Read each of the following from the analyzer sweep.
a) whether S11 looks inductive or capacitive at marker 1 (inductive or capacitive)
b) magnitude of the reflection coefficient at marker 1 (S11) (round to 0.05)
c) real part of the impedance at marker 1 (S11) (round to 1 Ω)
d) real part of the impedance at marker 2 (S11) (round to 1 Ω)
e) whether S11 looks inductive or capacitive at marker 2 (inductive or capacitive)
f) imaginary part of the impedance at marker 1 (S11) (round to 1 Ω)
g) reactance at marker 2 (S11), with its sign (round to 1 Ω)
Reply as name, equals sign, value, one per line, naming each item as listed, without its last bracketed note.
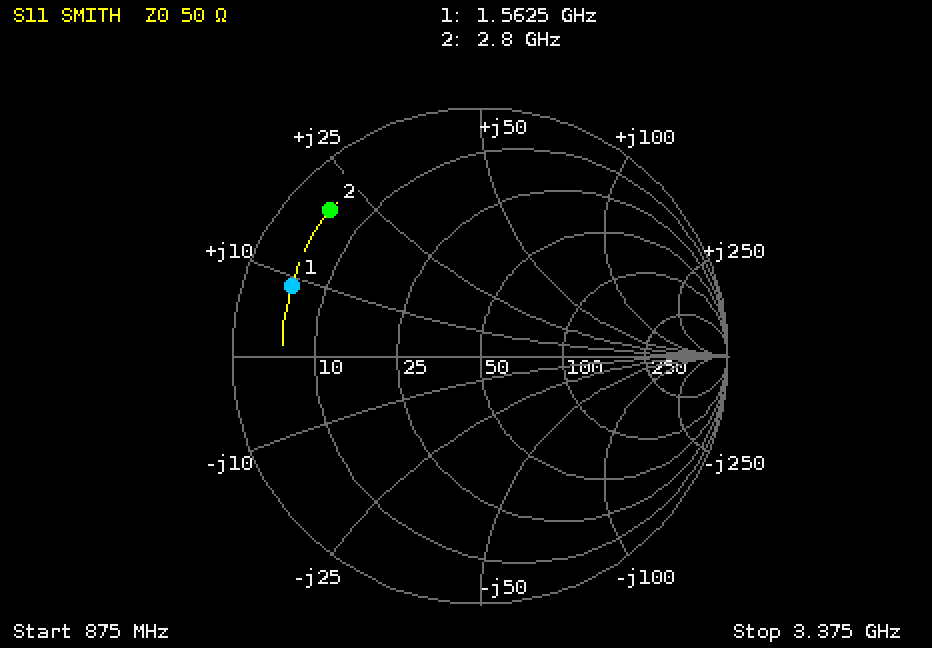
whether S11 looks inductive or capacitive at marker 1 = inductive
magnitude of the reflection coefficient at marker 1 (S11) = 0.80
real part of the impedance at marker 1 (S11) = 5 Ω
real part of the impedance at marker 2 (S11) = 5 Ω
whether S11 looks inductive or capacitive at marker 2 = inductive
imaginary part of the impedance at marker 1 (S11) = +9 Ω
reactance at marker 2 (S11), with its sign = +20 Ω
